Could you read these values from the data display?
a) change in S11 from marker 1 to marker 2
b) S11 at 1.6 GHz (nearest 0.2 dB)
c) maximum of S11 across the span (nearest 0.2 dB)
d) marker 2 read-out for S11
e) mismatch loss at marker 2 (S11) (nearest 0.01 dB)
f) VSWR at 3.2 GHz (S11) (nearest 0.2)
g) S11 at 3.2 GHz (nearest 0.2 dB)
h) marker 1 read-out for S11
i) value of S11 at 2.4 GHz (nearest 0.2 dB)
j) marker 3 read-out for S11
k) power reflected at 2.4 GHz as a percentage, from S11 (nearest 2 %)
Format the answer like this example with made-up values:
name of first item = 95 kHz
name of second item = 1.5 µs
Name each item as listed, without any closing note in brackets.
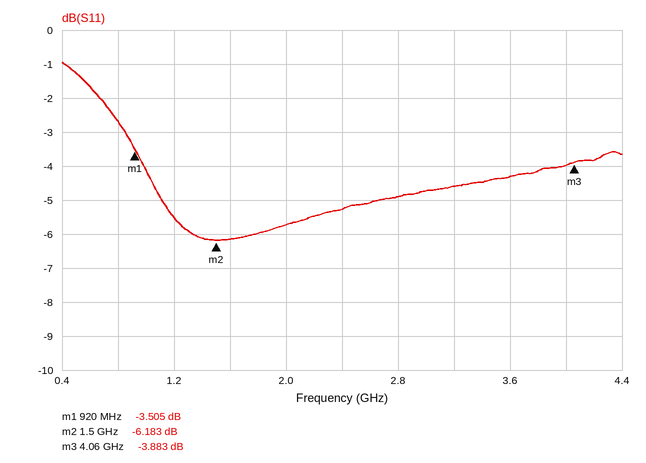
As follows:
change in S11 from marker 1 to marker 2 = -2.678 dB
S11 at 1.6 GHz = -6.2 dB
maximum of S11 across the span = -1.0 dB
marker 2 read-out for S11 = -6.183 dB
mismatch loss at marker 2 (S11) = 1.20 dB
VSWR at 3.2 GHz (S11) = 3.8
S11 at 3.2 GHz = -4.6 dB
marker 1 read-out for S11 = -3.505 dB
value of S11 at 2.4 GHz = -5.2 dB
marker 3 read-out for S11 = -3.883 dB
power reflected at 2.4 GHz as a percentage, from S11 = 30 %
